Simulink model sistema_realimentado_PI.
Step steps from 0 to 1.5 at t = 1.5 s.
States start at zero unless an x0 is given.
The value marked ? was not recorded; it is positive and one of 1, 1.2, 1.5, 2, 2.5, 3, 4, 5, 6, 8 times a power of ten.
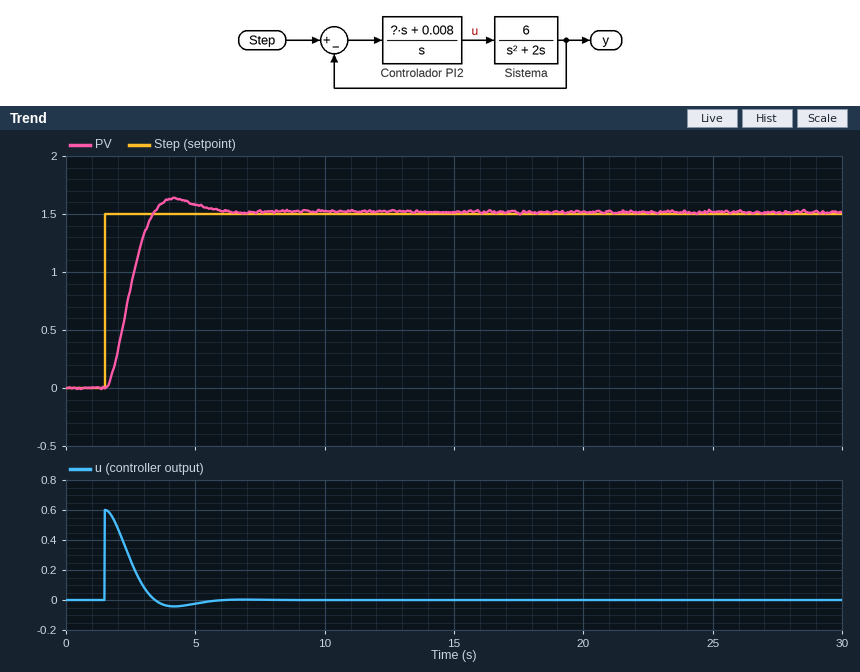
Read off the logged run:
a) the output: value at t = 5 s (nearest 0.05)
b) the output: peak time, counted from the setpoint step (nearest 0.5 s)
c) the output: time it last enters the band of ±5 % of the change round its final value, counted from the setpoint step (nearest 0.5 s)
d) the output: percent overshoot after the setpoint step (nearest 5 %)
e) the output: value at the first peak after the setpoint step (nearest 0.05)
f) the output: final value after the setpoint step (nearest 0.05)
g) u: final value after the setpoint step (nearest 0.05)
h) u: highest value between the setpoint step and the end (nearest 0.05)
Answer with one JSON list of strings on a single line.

["1.60", "2.5 s", "3.5 s", "10 %", "1.65", "1.50", "0.00", "0.60"]
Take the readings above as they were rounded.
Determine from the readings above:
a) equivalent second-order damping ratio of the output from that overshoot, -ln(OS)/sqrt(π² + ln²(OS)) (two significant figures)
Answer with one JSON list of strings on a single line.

["0.59"]
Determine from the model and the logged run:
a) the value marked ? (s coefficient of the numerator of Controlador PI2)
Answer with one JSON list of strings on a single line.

["0.4"]
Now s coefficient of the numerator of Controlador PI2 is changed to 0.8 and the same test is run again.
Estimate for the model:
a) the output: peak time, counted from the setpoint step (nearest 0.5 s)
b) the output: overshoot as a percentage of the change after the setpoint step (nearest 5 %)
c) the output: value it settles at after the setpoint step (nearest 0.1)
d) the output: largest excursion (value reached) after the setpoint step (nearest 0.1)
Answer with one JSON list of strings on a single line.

["1.5 s", "20 %", "1.5", "1.8"]
